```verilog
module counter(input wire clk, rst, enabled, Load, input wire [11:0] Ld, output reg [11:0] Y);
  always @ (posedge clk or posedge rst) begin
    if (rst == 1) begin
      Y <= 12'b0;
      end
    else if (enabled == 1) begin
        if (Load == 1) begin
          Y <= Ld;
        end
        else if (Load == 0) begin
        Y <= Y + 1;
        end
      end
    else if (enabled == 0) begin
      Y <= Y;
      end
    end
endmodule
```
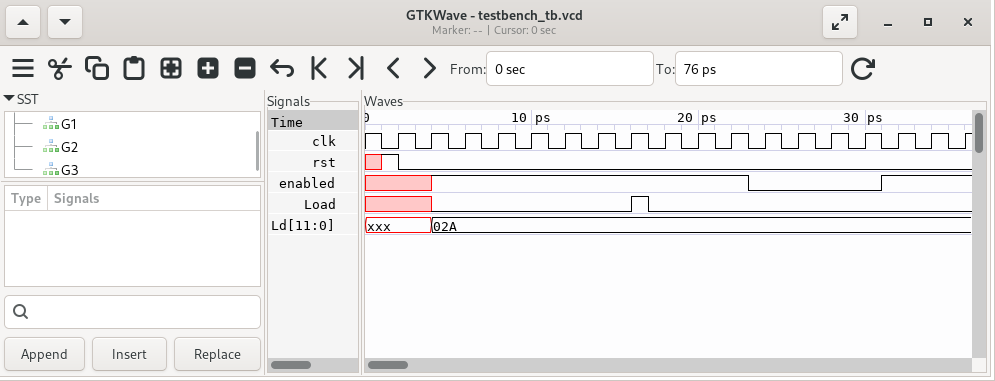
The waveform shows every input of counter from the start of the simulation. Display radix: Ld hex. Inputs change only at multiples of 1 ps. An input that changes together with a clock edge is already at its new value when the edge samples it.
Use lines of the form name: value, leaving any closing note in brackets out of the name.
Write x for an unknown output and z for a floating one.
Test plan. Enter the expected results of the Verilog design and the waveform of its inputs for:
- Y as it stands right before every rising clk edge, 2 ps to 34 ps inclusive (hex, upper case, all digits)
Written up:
Y as it stands right before every rising clk edge, 2 ps to 34 ps inclusive: 000, 000, 001, 002, 003, 004, 005, 006, 02A, 02B, 02C, 02D, 02D, 02D, 02D, 02D, 02E
